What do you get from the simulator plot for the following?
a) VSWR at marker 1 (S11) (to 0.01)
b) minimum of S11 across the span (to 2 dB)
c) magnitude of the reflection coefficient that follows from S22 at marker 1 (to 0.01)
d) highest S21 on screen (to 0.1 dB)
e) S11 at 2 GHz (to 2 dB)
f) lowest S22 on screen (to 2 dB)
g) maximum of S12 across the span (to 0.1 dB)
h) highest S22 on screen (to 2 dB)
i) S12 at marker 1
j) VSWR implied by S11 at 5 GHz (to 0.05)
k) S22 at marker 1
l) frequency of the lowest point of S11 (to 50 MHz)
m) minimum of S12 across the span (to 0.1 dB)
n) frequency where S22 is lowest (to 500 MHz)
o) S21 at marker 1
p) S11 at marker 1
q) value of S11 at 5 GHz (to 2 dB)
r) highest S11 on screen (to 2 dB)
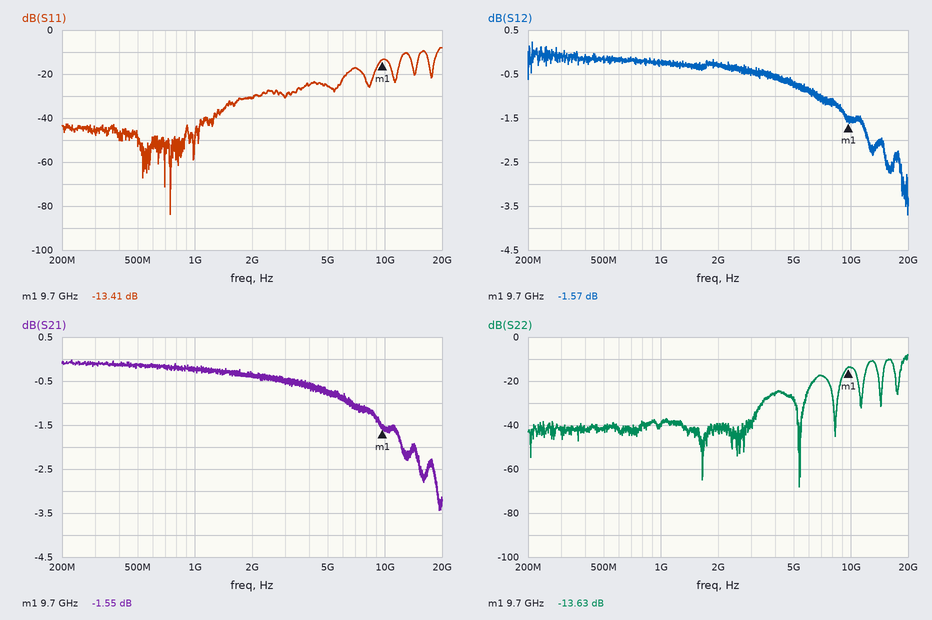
1.54
-84 dB
0.21
0.0 dB
-30 dB
-68 dB
0.2 dB
-8 dB
-1.57 dB
1.10
-13.63 dB
750 MHz
-3.7 dB
5.5 GHz
-1.55 dB
-13.41 dB
-26 dB
-8 dB
